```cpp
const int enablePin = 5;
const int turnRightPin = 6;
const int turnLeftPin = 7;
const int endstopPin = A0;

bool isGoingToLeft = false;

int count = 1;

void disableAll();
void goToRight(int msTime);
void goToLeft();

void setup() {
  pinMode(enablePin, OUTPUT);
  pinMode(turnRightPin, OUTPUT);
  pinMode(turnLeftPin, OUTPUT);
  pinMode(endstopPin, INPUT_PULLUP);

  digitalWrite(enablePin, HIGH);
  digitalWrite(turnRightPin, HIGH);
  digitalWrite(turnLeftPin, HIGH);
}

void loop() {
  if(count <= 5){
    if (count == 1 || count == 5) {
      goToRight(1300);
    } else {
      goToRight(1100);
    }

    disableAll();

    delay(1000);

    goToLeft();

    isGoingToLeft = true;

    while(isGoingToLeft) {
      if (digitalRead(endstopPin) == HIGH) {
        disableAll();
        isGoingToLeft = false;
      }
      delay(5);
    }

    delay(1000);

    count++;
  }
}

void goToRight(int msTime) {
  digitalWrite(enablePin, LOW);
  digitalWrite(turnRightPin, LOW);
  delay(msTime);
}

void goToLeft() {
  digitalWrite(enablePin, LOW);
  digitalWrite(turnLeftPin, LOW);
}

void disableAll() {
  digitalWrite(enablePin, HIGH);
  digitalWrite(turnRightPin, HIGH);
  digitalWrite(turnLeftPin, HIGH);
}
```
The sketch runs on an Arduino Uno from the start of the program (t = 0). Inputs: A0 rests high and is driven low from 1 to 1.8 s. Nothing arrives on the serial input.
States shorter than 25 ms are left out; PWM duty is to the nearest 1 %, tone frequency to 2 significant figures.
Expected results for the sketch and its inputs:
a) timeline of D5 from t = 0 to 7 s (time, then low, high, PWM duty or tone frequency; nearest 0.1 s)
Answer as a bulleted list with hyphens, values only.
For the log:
- 0 s low; 1.3 s high; 3.3 s low; 4.4 s high; 6.4 s low
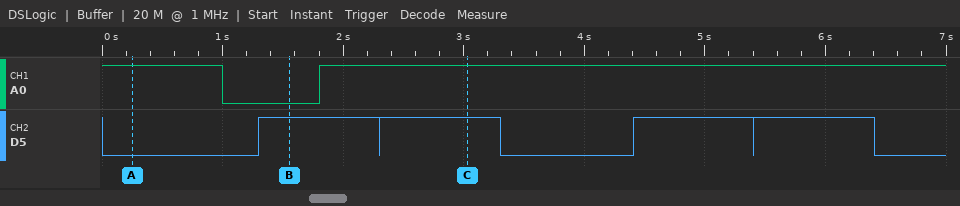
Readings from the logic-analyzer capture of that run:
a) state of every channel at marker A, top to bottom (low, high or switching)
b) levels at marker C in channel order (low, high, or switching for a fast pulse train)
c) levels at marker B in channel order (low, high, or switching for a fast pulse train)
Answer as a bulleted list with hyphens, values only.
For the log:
- A0 high, D5 low
- A0 high, D5 high
- A0 low, D5 high
